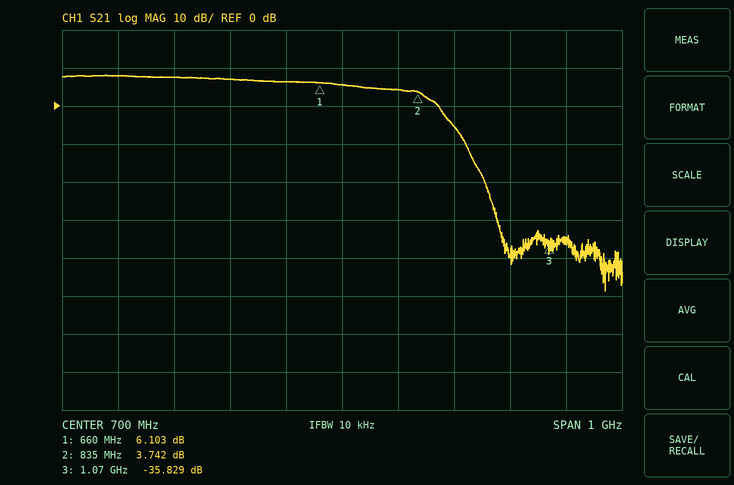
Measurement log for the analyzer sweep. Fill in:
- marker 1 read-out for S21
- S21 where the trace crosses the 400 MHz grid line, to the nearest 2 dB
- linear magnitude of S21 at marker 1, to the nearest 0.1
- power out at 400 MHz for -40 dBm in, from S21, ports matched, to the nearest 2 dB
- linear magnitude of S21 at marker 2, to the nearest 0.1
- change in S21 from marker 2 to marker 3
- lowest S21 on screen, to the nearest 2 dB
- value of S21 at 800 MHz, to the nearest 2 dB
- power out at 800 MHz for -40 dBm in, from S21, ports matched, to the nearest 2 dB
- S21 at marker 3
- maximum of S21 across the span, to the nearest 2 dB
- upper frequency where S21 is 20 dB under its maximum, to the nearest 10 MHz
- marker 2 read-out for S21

6.103 dB
8 dB
2.0
-32 dBm
1.5
-39.571 dB
-48 dB
4 dB
-36 dBm
-35.829 dB
8 dB
930 MHz
3.742 dB
